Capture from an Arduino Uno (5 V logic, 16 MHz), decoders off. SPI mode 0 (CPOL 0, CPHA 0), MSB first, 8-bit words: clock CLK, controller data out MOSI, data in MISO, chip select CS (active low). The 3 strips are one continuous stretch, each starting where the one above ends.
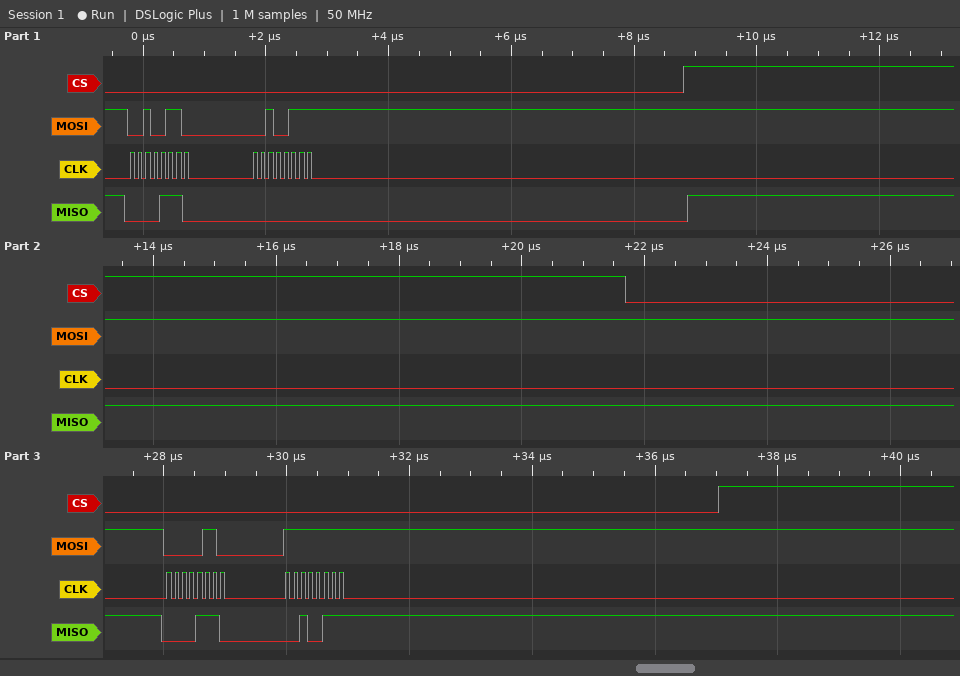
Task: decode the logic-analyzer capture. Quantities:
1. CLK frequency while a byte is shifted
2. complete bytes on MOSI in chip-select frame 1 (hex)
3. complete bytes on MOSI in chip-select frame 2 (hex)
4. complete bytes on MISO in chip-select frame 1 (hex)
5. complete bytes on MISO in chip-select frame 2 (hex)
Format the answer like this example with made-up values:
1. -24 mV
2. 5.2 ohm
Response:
1. 8 MHz
2. 0x26 0x27
3. 0x06 0xFF
4. 0x0E 0x00
5. 0x0E 0x27
